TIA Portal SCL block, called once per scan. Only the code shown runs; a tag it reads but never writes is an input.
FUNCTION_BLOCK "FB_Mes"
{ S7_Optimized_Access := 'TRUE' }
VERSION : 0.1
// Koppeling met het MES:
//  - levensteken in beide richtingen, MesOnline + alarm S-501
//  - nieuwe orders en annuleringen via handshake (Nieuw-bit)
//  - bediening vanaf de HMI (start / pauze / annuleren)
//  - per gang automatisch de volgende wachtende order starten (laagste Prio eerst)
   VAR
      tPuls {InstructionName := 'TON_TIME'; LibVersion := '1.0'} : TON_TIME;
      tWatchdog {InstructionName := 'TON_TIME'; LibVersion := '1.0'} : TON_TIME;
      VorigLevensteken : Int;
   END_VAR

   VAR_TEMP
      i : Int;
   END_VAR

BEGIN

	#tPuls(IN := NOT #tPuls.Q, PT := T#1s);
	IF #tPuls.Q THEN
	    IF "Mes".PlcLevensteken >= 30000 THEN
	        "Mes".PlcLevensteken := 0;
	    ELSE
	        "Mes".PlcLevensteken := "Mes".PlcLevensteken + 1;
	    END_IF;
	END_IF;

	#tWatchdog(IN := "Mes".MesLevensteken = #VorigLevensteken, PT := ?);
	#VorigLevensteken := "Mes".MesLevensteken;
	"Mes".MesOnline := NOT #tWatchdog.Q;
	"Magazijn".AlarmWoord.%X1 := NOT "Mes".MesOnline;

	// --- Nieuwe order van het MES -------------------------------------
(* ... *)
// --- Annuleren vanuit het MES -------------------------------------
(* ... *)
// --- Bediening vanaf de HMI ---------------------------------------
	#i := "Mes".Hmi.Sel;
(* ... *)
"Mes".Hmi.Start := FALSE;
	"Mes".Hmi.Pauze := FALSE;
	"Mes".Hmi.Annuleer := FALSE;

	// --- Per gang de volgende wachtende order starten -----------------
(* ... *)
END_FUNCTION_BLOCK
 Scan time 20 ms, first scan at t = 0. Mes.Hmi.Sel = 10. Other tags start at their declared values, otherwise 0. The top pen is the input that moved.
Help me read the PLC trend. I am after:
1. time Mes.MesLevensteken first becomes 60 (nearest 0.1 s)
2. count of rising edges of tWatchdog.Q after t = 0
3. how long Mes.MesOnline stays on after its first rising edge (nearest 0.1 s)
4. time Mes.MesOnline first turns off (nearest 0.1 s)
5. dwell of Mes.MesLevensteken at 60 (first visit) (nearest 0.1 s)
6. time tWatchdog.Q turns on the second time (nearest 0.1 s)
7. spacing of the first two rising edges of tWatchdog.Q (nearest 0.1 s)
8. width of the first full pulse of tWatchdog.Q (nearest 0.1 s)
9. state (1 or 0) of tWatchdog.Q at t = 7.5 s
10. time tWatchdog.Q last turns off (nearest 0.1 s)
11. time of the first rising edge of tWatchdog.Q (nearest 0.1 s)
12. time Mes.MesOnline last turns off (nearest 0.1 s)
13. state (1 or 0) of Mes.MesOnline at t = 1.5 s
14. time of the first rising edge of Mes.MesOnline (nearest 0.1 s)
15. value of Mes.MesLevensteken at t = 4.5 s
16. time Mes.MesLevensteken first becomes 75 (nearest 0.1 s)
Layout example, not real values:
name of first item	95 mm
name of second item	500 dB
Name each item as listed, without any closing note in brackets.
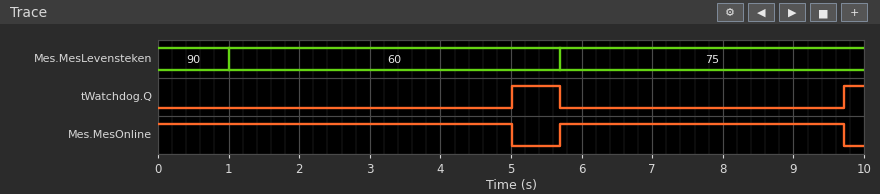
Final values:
time Mes.MesLevensteken first becomes 60	1.0 s
count of rising edges of tWatchdog.Q after t = 0	2
how long Mes.MesOnline stays on after its first rising edge	4.0 s
time Mes.MesOnline first turns off	5.0 s
dwell of Mes.MesLevensteken at 60 (first visit)	4.7 s
time tWatchdog.Q turns on the second time	9.7 s
spacing of the first two rising edges of tWatchdog.Q	4.7 s
width of the first full pulse of tWatchdog.Q	0.7 s
state (1 or 0) of tWatchdog.Q at t = 7.5 s	0
time tWatchdog.Q last turns off	5.7 s
time of the first rising edge of tWatchdog.Q	5.0 s
time Mes.MesOnline last turns off	9.7 s
state (1 or 0) of Mes.MesOnline at t = 1.5 s	1
time of the first rising edge of Mes.MesOnline	5.7 s
value of Mes.MesLevensteken at t = 4.5 s	60
time Mes.MesLevensteken first becomes 75	5.7 s
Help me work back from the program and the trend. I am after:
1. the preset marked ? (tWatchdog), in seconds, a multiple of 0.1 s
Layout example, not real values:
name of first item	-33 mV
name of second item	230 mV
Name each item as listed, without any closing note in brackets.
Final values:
the preset marked ? (tWatchdog), in seconds, a multiple of 0.1 s	4.0 s
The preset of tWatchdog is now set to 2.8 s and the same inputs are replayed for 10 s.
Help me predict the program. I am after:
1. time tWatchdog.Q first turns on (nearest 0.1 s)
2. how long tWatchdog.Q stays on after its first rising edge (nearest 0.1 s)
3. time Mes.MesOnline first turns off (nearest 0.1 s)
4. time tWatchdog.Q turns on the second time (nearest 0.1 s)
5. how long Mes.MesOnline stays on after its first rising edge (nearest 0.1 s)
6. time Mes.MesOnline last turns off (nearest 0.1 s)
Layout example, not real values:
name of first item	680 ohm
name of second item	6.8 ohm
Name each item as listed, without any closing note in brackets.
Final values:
time tWatchdog.Q first turns on	3.8 s
how long tWatchdog.Q stays on after its first rising edge	1.9 s
time Mes.MesOnline first turns off	3.8 s
time tWatchdog.Q turns on the second time	8.5 s
how long Mes.MesOnline stays on after its first rising edge	2.8 s
time Mes.MesOnline last turns off	8.5 s
